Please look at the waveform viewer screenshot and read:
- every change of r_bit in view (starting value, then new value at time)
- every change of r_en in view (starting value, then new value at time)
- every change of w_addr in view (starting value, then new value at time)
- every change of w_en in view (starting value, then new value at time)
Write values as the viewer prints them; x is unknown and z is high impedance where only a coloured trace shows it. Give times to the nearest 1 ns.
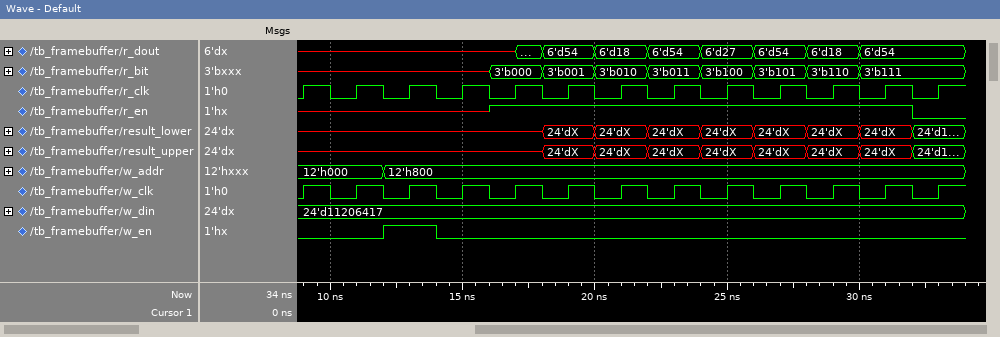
x, 3'b000 at 16 ns, 3'b001 at 18 ns, 3'b010 at 20 ns, 3'b011 at 22 ns, 3'b100 at 24 ns, 3'b101 at 26 ns, 3'b110 at 28 ns, 3'b111 at 30 ns
x, 1 at 16 ns, 0 at 32 ns
12'h000, 12'h800 at 12 ns
0, 1 at 12 ns, 0 at 14 ns
